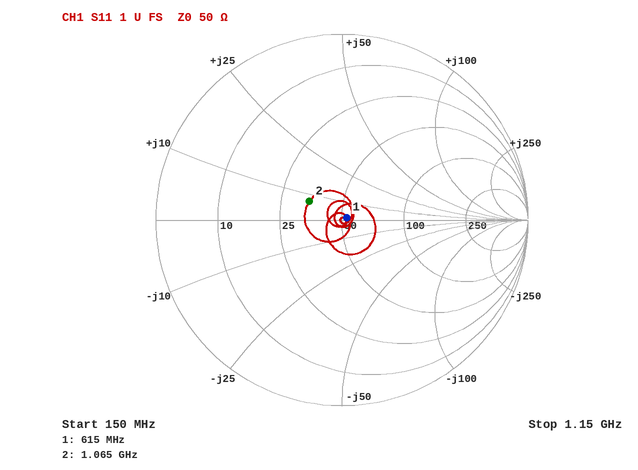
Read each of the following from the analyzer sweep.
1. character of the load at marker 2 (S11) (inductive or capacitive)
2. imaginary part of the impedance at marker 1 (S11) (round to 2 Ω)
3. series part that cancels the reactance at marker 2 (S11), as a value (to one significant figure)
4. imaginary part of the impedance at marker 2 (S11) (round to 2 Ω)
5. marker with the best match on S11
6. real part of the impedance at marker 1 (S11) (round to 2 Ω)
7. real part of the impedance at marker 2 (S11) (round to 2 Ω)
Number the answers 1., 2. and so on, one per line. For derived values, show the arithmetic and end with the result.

1. inductive
2. +2 Ω
3. C = 1/(2π × 1.065 GHz × 8 Ω) ≈ 18.7 pF, so 20 pF to one significant figure
4. +8 Ω
5. marker 1
6. 52 Ω
7. 34 Ω
